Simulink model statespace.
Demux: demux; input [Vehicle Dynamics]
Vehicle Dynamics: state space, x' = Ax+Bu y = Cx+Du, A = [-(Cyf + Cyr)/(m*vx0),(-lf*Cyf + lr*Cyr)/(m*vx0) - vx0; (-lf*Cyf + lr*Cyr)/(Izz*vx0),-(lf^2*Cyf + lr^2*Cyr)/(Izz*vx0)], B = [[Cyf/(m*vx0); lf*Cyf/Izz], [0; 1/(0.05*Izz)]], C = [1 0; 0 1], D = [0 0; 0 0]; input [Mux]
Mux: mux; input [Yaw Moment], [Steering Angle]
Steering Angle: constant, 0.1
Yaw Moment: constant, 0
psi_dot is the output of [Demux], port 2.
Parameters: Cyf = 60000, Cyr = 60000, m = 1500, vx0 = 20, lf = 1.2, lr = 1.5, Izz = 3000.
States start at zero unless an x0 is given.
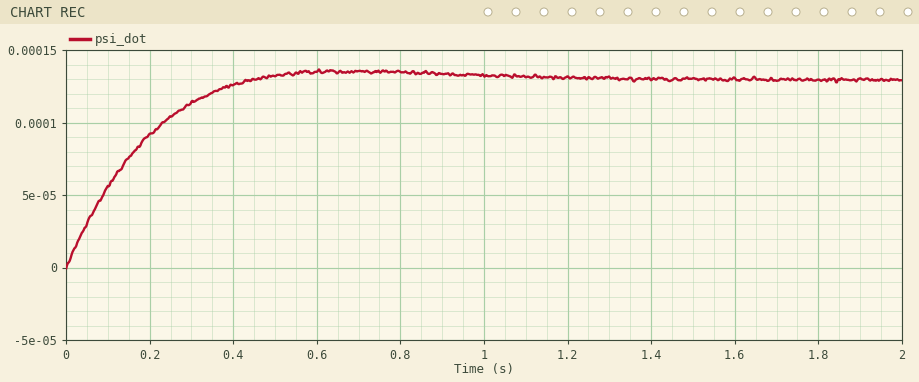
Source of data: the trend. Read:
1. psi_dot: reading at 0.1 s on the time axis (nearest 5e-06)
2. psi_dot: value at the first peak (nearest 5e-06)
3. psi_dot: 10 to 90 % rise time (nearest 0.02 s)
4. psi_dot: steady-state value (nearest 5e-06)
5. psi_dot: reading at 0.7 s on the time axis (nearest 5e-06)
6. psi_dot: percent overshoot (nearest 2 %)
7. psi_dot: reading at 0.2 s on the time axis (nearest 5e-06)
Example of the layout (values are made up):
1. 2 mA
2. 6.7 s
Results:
1. 0.000055
2. 0.000135
3. 0.30 s
4. 0.000130
5. 0.000135
6. 4 %
7. 0.000090
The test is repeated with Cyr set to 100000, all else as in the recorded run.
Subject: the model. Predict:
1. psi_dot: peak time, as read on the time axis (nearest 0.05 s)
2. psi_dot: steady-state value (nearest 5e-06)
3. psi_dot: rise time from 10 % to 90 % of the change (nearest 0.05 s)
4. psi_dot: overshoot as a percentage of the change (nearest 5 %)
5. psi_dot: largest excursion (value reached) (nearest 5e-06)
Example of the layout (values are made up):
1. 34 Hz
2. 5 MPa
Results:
1. 0.35 s
2. 0.000070
3. 0.15 s
4. 15 %
5. 0.000080
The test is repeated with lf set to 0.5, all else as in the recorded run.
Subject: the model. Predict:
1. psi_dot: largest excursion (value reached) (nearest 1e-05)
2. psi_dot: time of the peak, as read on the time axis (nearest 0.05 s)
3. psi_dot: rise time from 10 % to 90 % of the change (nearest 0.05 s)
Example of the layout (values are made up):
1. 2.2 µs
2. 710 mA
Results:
1. 0.00012
2. 0.40 s
3. 0.15 s
